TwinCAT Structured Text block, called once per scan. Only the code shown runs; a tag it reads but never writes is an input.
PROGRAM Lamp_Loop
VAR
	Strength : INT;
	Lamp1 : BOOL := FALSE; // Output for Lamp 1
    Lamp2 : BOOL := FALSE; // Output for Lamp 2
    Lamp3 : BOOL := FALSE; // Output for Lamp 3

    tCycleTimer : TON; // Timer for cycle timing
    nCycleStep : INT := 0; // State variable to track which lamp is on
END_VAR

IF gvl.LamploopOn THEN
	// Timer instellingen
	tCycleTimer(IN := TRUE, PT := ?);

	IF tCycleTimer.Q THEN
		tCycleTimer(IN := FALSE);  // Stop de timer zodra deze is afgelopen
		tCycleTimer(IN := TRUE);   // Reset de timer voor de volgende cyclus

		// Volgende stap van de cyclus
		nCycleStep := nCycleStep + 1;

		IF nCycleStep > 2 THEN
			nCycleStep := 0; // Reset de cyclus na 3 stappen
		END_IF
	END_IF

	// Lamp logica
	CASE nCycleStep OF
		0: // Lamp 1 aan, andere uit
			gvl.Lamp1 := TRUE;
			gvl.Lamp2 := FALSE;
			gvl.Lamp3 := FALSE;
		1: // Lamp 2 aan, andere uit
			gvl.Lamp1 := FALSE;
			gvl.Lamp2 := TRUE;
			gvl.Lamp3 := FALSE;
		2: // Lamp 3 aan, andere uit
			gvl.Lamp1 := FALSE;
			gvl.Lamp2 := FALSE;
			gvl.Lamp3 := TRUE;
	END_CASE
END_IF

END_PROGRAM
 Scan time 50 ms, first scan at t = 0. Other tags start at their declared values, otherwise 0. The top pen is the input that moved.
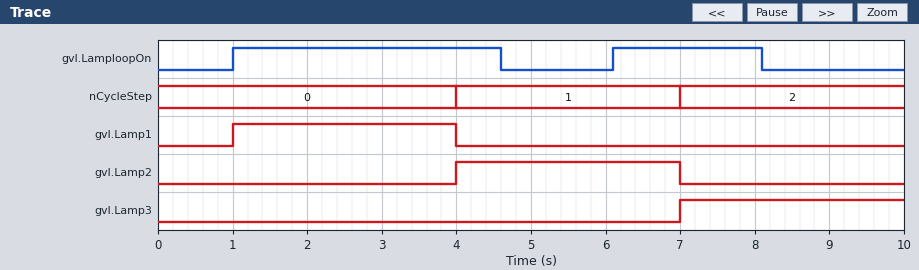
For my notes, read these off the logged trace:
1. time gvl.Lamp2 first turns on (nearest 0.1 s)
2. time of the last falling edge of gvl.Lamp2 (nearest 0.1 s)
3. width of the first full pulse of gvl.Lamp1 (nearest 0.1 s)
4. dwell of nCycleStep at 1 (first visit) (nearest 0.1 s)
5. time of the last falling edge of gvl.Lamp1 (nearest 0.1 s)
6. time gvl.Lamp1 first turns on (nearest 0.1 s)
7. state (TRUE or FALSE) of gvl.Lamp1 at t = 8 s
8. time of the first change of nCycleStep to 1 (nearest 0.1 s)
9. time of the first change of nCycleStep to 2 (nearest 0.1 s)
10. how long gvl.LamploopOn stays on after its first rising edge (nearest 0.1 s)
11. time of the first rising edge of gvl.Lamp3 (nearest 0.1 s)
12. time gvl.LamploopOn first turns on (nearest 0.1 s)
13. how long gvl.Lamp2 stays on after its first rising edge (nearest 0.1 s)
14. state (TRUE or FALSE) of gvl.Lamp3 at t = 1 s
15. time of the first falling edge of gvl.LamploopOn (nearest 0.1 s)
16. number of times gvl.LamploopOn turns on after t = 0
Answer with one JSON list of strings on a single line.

["4.0 s", "7.0 s", "3.0 s", "3.0 s", "4.0 s", "1.0 s", "FALSE", "4.0 s", "7.0 s", "3.6 s", "7.0 s", "1.0 s", "3.0 s", "FALSE", "4.6 s", "2"]
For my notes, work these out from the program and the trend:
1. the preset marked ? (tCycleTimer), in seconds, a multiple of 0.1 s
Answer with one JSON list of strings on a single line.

["3.0 s"]
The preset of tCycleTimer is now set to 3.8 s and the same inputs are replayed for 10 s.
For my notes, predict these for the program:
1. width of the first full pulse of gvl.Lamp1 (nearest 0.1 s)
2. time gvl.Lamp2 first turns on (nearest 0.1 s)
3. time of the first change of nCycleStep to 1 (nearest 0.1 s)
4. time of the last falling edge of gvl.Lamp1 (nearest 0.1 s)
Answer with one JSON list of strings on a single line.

["5.1 s", "6.1 s", "6.1 s", "6.1 s"]
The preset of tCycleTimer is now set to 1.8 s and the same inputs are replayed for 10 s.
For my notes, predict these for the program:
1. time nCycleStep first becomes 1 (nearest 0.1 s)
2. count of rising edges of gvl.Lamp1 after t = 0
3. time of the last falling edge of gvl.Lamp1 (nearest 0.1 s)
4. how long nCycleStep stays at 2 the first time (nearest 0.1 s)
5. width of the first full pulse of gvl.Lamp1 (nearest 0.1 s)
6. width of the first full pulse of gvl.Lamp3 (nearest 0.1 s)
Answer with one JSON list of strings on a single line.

["2.8 s", "2", "2.8 s", "1.8 s", "1.8 s", "1.8 s"]
